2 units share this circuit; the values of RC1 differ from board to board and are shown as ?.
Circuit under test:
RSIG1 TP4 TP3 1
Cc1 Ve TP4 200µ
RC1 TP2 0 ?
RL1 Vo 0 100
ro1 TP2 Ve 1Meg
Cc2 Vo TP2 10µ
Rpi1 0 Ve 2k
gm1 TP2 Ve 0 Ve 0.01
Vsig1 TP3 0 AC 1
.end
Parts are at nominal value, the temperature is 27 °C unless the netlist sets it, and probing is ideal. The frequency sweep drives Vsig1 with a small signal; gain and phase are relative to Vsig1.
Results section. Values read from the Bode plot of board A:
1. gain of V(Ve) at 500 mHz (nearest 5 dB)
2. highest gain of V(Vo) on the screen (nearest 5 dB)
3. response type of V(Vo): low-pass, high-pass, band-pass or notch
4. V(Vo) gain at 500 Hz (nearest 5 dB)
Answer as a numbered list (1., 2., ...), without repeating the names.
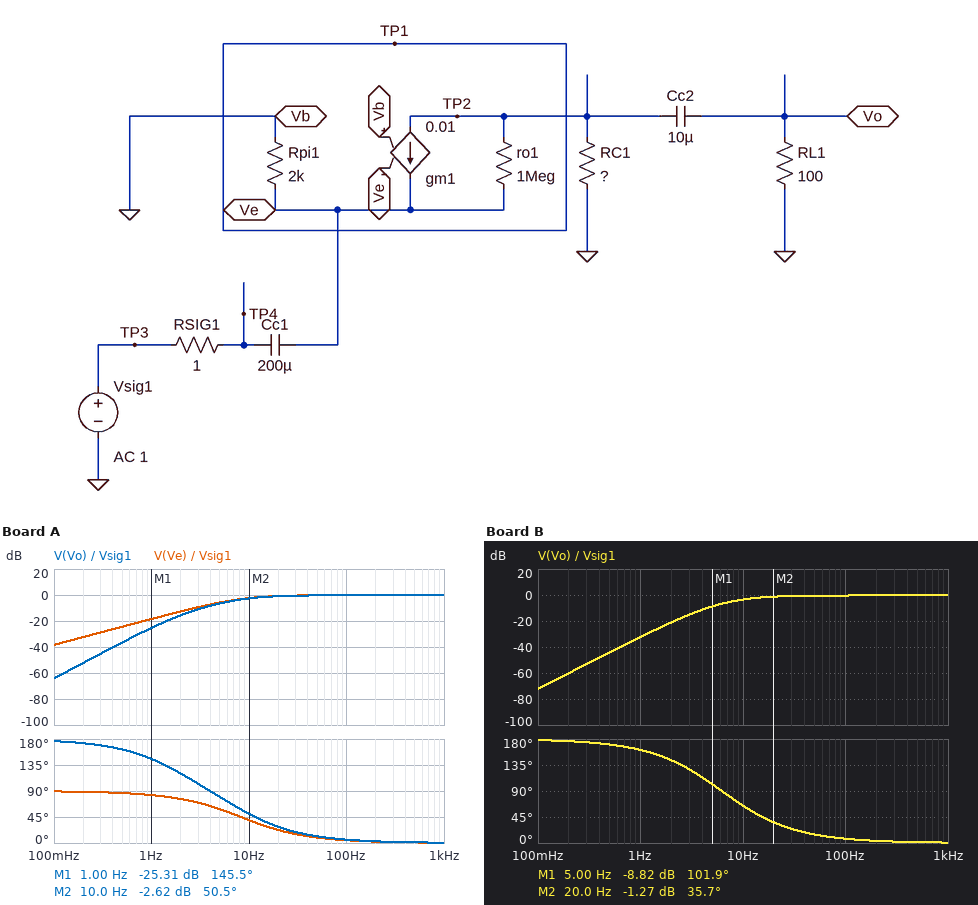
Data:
1. -25 dB
2. 0 dB
3. high-pass
4. 0 dB
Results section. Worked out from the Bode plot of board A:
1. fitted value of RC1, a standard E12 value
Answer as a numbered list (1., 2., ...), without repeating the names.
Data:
1. 8.2 kΩ
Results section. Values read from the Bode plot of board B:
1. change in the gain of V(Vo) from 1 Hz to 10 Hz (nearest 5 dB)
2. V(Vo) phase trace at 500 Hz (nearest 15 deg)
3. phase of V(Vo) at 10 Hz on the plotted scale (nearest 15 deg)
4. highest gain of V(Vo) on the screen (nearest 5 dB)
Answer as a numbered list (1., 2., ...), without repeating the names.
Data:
1. 30 dB
2. 0 deg
3. 60 deg
4. 0 dB
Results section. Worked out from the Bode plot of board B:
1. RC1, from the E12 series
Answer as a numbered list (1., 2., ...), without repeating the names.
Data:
1. 3.3 kΩ
